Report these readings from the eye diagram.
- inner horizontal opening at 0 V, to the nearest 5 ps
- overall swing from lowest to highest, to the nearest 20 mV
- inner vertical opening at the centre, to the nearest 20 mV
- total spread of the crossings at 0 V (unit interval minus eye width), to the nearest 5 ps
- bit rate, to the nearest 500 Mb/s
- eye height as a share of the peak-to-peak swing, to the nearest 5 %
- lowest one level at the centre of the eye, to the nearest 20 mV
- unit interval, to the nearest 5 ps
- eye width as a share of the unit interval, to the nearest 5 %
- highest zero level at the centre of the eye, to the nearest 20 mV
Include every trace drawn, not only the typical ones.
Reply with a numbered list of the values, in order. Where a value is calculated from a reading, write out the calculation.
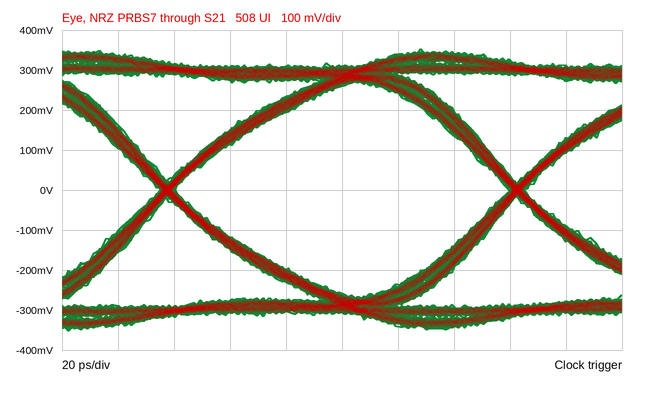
1. 120 ps
2. 700 mV
3. 520 mV
4. 5 ps
5. 8.0 Gb/s
6. 520 mV / 700 mV ≈ 74.3 %, so 75 % to the nearest 5 %
7. 260 mV
8. 125 ps
9. 120 ps / 125 ps ≈ 96.0 %, so 95 % to the nearest 5 %
10. -260 mV
